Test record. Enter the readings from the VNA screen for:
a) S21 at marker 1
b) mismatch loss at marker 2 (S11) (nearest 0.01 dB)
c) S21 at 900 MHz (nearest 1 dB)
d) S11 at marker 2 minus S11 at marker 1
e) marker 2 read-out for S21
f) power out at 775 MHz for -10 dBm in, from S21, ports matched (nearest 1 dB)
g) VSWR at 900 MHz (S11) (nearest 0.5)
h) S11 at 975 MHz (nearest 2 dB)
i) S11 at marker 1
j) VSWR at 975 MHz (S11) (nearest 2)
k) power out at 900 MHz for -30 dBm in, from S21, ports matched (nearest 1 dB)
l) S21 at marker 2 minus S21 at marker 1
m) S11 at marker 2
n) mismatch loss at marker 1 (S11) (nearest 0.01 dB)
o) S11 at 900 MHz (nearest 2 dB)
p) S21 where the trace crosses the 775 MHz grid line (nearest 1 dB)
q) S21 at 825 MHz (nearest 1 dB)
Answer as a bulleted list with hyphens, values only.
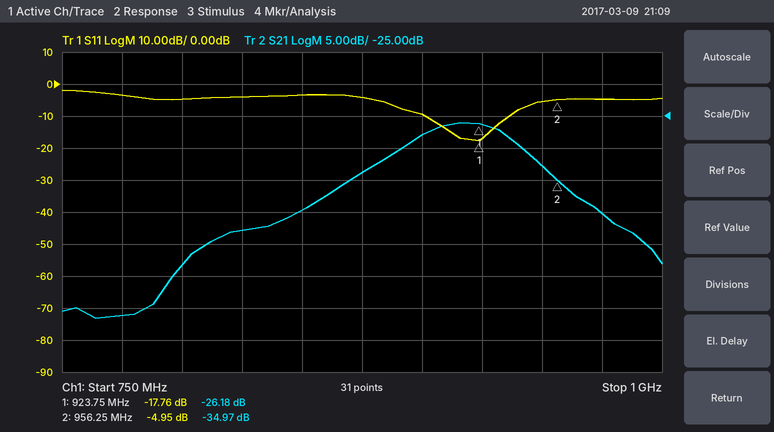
- -26.18 dB
- 1.67 dB
- -28 dB
- 12.81 dB
- -34.97 dB
- -66 dBm
- 2.0
- -4 dB
- -17.76 dB
- 4
- -58 dBm
- -8.79 dB
- -4.95 dB
- 0.07 dB
- -10 dB
- -56 dB
- -43 dB
